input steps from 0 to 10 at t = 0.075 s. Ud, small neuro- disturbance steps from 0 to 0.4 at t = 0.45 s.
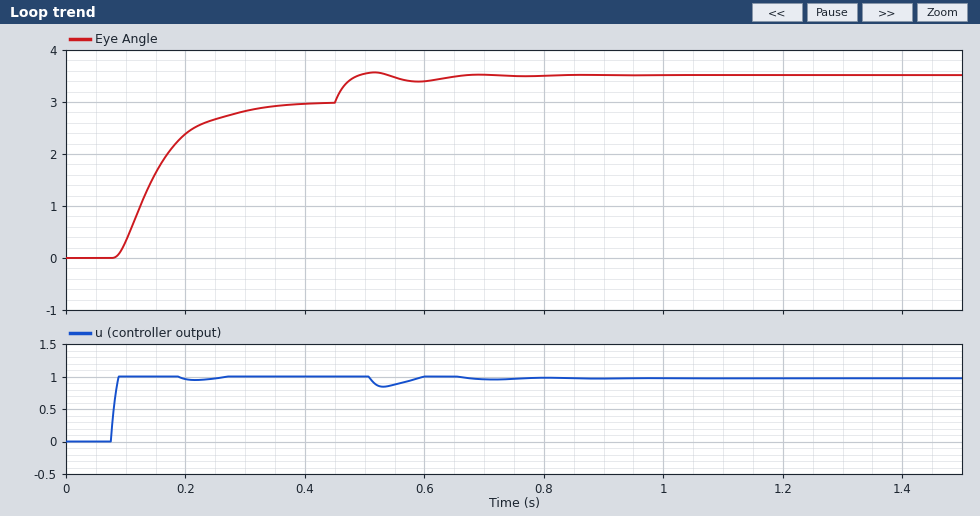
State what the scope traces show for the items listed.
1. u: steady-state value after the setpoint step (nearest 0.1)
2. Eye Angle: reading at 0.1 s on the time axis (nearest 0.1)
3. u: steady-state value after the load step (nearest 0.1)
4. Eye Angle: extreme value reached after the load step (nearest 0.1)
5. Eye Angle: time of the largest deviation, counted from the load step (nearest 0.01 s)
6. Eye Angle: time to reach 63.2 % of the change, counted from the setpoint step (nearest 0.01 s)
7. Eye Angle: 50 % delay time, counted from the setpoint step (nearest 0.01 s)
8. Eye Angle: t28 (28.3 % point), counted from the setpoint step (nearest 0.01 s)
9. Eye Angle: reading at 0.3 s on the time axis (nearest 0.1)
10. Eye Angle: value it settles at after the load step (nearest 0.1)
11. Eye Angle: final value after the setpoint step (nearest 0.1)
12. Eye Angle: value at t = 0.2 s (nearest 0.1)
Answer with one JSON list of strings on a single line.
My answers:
["1.0", "0.3", "1.0", "3.6", "0.07 s", "0.09 s", "0.07 s", "0.04 s", "2.8", "3.5", "3.0", "2.4"]
